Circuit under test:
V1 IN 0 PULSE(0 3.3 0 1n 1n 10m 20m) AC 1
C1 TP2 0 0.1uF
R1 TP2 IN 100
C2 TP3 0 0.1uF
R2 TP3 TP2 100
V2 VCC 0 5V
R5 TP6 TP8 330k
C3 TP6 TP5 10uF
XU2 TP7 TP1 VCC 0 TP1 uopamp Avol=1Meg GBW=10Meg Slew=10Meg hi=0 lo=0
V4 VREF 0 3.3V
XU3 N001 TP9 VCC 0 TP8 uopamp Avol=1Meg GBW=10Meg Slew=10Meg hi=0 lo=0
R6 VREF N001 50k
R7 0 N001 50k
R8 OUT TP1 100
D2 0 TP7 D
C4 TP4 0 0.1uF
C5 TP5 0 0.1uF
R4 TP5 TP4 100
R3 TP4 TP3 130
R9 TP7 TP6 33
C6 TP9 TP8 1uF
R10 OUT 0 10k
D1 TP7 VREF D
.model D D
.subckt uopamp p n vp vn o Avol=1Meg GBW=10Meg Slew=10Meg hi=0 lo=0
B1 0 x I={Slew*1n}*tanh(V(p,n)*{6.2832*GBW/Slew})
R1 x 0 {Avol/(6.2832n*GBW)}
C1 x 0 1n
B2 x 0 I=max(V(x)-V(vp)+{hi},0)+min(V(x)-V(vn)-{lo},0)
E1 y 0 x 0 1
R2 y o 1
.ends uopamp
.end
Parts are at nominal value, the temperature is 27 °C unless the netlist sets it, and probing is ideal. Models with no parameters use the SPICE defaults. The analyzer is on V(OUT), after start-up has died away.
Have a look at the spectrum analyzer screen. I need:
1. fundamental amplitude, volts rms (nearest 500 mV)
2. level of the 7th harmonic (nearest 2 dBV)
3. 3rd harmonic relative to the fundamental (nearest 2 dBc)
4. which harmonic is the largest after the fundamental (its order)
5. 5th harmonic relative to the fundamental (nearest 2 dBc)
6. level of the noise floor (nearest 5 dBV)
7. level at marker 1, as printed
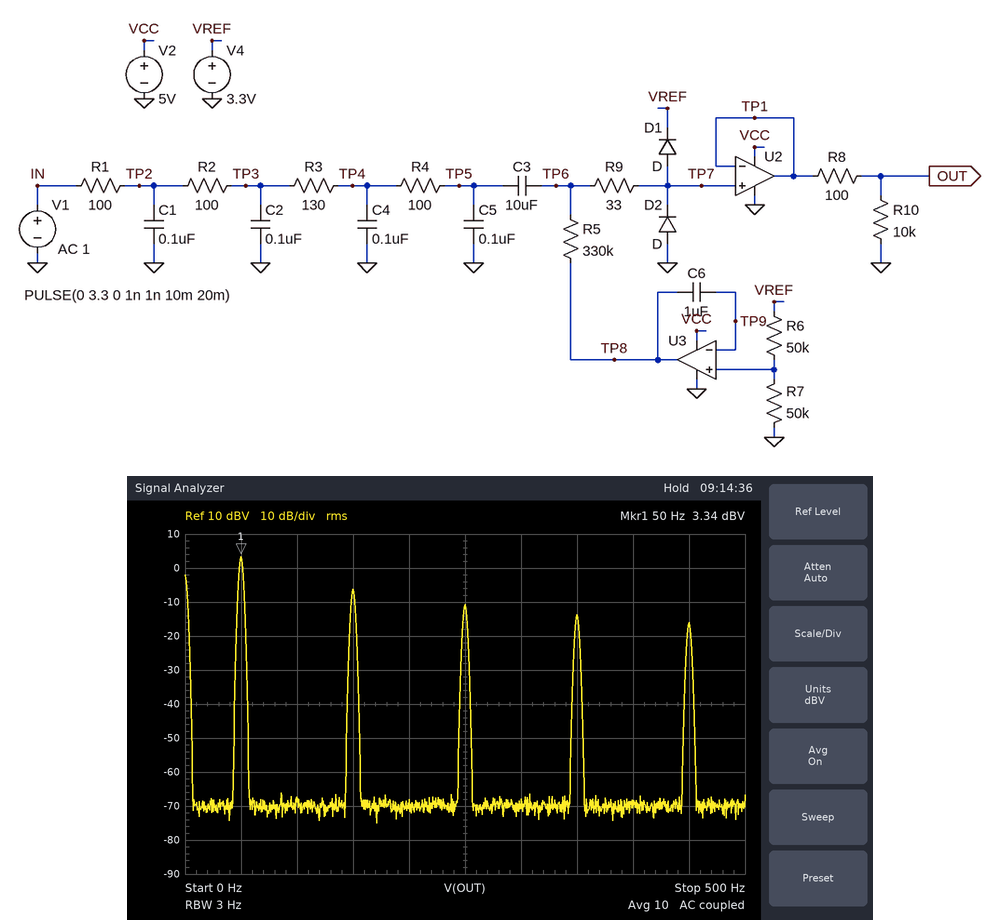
1.5 V
-14 dBV
-10 dBc
3
-14 dBc
-70 dBV
3.34 dBV
